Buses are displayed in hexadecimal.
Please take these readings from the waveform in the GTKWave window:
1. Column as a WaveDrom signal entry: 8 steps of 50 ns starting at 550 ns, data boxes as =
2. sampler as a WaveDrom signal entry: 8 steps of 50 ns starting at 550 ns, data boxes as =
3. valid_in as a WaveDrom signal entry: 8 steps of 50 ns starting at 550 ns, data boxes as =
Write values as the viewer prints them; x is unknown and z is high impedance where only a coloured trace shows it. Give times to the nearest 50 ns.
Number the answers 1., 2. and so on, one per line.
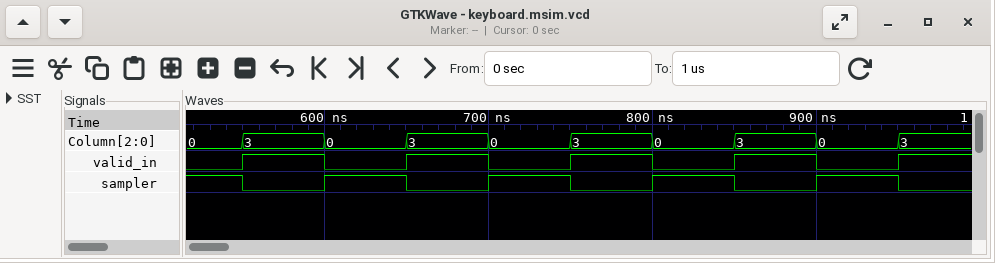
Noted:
1. {name: 'Column', wave: '========', data: '3 0 3 0 3 0 3 0'}
2. {name: 'sampler', wave: '01010101'}
3. {name: 'valid_in', wave: '10101010'}
